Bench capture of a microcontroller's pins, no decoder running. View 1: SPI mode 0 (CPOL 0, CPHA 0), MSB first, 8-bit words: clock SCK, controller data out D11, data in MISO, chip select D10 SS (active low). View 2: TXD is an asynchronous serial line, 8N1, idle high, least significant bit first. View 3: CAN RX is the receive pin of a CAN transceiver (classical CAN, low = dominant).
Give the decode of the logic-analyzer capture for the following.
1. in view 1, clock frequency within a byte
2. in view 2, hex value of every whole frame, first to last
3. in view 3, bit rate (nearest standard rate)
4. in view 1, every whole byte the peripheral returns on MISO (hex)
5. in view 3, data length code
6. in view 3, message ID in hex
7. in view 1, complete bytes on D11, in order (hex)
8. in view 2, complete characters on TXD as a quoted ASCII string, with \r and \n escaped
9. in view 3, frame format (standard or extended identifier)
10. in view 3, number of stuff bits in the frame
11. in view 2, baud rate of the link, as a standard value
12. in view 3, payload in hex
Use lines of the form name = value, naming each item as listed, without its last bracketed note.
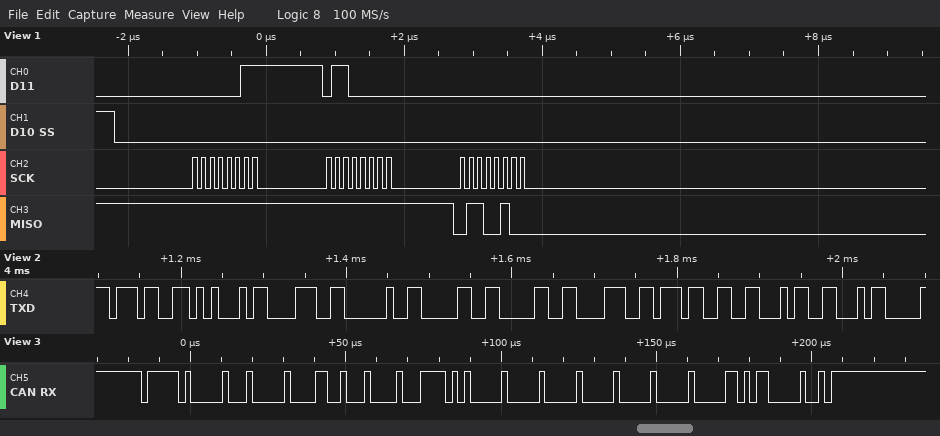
in view 1, clock frequency within a byte = 8 MHz
in view 2, hex value of every whole frame, first to last = 37 45 38 20 30 30 38 37 46 46
in view 3, bit rate = 500 kbit/s
in view 1, every whole byte the peripheral returns on MISO = 0xFF 0xFF 0x64
in view 3, data length code = 8
in view 3, message ID in hex = 0x7E0
in view 1, complete bytes on D11, in order = 0x03 0x60 0x00
in view 2, complete characters on TXD as a quoted ASCII string, with \r and \n escaped = "7E8 0087FF"
in view 3, frame format = standard
in view 3, number of stuff bits in the frame = 11
in view 2, baud rate of the link, as a standard value = 115200 baud
in view 3, payload in hex = 03 22 11 EA 00 00 00 00
